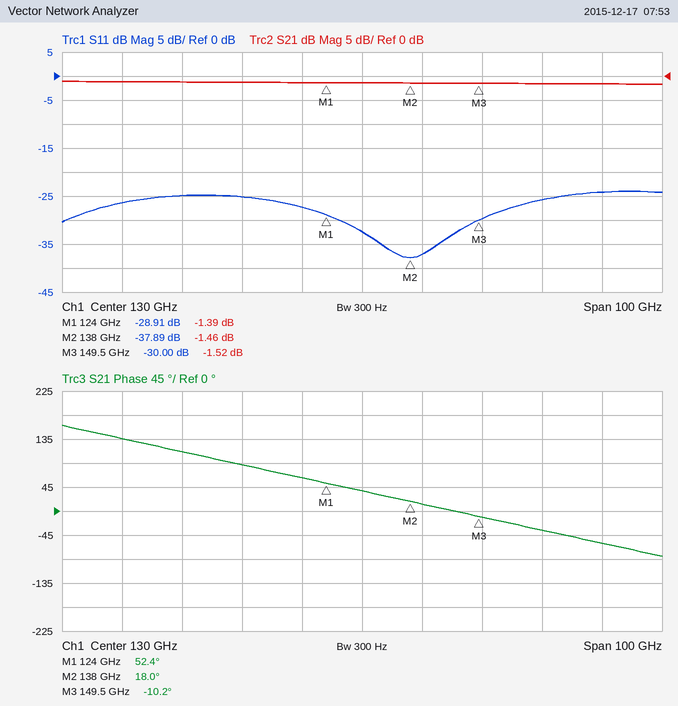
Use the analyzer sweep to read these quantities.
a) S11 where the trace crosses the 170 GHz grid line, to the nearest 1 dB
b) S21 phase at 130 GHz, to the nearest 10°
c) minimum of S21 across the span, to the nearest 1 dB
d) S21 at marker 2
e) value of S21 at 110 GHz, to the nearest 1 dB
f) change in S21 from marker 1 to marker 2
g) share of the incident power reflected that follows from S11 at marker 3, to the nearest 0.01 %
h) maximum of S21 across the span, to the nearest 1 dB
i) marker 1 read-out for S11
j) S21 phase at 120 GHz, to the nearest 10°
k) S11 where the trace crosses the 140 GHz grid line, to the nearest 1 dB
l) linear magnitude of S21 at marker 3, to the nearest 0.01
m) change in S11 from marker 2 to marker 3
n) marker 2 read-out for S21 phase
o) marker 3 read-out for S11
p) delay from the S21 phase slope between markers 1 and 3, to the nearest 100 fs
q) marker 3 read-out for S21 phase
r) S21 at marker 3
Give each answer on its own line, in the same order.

-24 dB
40°
-2 dB
-1.46 dB
-1 dB
-0.07 dB
0.10 %
-1 dB
-28.91 dB
60°
-37 dB
0.84
7.89 dB
18.0°
-30.00 dB
6.8 ps
-10.2°
-1.52 dB
